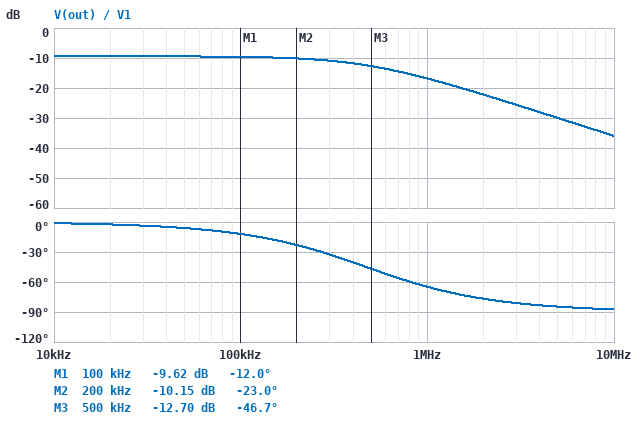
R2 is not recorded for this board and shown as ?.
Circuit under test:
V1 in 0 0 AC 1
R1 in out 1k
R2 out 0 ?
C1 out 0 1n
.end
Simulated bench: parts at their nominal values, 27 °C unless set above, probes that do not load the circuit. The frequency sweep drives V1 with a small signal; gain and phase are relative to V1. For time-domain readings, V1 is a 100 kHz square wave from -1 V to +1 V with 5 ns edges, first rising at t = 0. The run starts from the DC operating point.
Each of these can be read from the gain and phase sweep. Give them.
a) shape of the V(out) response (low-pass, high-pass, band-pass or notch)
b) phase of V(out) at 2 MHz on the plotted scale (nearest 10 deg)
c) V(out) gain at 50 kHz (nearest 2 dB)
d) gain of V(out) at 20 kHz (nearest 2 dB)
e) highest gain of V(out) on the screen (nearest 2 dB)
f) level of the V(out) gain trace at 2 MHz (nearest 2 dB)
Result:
low-pass
-80 deg
-10 dB
-10 dB
-10 dB
-22 dB
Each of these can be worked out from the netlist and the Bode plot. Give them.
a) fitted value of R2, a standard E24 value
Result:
510 Ω
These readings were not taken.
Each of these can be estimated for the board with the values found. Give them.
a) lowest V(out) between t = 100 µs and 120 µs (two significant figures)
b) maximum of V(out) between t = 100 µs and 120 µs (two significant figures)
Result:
-340 mV
340 mV
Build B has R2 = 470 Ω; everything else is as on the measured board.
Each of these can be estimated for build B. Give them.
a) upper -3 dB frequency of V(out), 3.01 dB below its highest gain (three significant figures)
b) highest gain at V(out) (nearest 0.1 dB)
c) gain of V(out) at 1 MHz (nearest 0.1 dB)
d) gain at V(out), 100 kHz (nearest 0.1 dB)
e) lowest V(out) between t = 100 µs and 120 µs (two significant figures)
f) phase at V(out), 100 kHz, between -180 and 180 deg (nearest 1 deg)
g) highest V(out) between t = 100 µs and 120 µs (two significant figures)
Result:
498 kHz
-9.9 dB
-16.9 dB
-10.1 dB
-320 mV
-11 deg
320 mV
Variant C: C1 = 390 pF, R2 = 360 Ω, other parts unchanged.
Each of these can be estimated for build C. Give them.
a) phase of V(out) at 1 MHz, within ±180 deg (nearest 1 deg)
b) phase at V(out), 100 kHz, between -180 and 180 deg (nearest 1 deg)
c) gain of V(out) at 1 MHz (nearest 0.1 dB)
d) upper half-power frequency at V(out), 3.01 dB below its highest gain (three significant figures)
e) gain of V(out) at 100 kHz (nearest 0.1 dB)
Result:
-33 deg
-4 deg
-13.1 dB
1.54 MHz
-11.6 dB
